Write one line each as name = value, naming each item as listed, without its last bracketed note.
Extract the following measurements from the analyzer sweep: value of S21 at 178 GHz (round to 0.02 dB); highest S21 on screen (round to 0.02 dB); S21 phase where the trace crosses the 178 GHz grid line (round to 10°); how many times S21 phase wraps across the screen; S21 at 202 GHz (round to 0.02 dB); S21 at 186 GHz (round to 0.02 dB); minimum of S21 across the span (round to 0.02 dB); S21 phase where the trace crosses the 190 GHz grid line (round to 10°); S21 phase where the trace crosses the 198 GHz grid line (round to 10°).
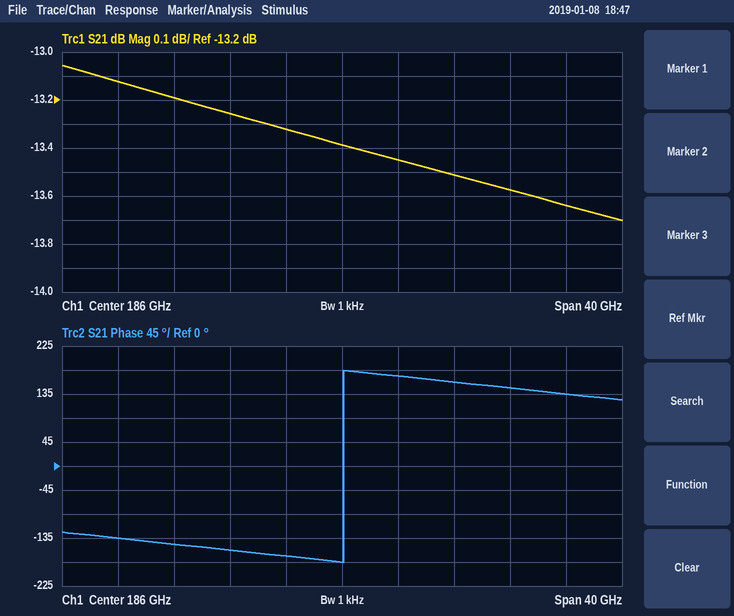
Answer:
value of S21 at 178 GHz = -13.26 dB
highest S21 on screen = -13.06 dB
S21 phase where the trace crosses the 178 GHz grid line = -160°
how many times S21 phase wraps across the screen = 1
S21 at 202 GHz = -13.64 dB
S21 at 186 GHz = -13.38 dB
minimum of S21 across the span = -13.70 dB
S21 phase where the trace crosses the 190 GHz grid line = 170°
S21 phase where the trace crosses the 198 GHz grid line = 150°
